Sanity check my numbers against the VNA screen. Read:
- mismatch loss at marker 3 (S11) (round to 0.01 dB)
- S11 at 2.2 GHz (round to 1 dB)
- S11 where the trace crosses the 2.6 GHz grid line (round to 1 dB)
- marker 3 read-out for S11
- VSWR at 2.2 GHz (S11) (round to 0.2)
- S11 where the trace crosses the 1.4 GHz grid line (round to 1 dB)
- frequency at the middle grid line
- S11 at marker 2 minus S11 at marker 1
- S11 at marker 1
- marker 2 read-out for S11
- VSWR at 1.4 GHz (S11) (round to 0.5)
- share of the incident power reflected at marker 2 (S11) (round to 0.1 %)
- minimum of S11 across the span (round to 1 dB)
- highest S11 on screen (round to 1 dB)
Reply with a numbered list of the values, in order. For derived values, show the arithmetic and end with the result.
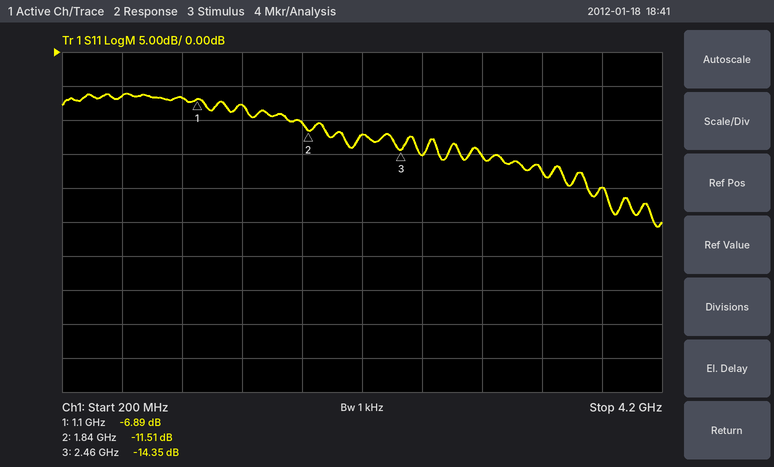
1. −10 log10(1 − 10^(-14.35/10)) ≈ 0.16 dB
2. -12 dB
3. -15 dB
4. -14.35 dB
5. |Γ| = 10^(-12/20) = 0.2512; VSWR = (1 + 0.2512)/(1 − 0.2512) ≈ 1.67, so 1.6 to the nearest 0.2
6. -8 dB
7. 2.2 GHz
8. -11.51 − (-6.89) = -4.62 dB
9. -6.89 dB
10. -11.51 dB
11. |Γ| = 10^(-8/20) = 0.3981; VSWR = (1 + 0.3981)/(1 − 0.3981) ≈ 2.32, so 2.5 to the nearest 0.5
12. 10^(-11.51/10) ≈ 7.1 %
13. -26 dB
14. -6 dB
